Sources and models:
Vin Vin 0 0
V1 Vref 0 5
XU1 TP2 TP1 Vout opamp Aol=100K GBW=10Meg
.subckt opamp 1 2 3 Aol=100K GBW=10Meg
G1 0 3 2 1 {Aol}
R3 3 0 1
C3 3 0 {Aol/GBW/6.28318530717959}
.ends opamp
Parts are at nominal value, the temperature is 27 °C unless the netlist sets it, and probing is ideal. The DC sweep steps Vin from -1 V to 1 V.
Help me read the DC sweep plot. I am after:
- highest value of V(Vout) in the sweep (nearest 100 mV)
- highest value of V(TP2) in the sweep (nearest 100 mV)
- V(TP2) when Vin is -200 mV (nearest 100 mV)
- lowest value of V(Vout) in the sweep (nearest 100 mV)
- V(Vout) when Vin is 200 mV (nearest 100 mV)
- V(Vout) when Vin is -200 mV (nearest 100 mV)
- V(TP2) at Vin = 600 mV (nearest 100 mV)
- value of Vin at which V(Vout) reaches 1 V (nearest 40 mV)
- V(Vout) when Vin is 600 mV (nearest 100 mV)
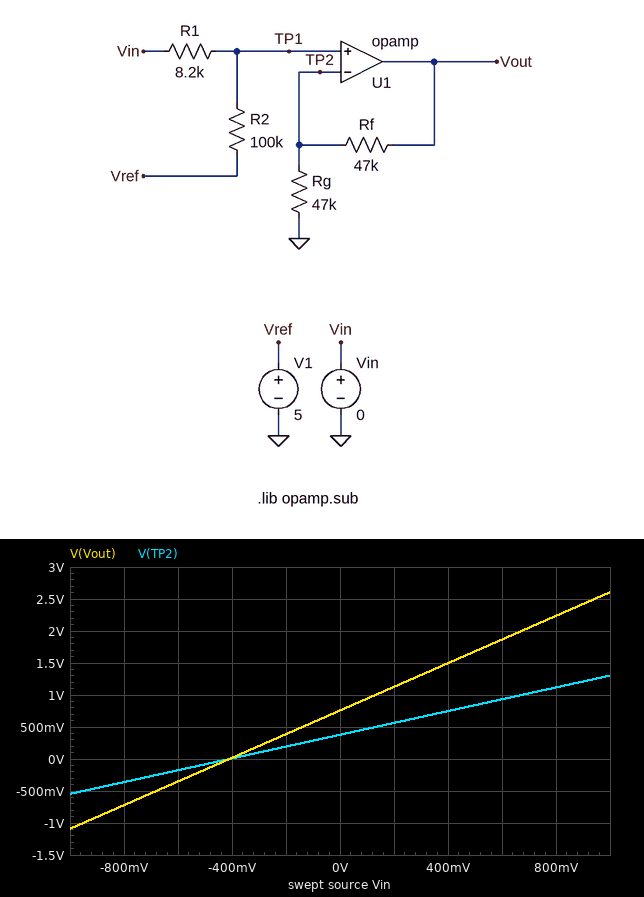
2.6 V
1.3 V
200 mV
-1.1 V
1.1 V
400 mV
900 mV
120 mV
1.9 V
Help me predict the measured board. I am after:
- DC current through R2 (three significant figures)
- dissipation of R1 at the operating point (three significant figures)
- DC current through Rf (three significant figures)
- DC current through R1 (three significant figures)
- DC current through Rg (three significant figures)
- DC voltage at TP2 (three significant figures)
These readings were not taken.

46.2 µA
17.5 µW
8.06 µA
46.2 µA
8.06 µA
379 mV
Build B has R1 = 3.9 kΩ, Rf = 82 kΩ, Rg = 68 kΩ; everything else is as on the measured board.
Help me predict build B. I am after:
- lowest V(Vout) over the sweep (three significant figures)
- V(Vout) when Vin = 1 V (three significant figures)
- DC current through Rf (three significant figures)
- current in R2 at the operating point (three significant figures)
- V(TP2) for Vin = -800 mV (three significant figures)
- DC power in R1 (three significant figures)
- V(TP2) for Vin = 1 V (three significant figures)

-1.71 V
2.54 V
2.76 µA
48.1 µA
-582 mV
9.03 µW
1.15 V
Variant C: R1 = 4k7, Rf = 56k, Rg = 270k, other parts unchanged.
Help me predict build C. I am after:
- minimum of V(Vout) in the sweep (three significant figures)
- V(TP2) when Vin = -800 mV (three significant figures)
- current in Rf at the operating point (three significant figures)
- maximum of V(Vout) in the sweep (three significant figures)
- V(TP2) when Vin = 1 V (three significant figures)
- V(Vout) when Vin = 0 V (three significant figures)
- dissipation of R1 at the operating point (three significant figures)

-882 mV
-540 mV
831 nA
1.42 V
1.18 V
271 mV
10.7 µW
